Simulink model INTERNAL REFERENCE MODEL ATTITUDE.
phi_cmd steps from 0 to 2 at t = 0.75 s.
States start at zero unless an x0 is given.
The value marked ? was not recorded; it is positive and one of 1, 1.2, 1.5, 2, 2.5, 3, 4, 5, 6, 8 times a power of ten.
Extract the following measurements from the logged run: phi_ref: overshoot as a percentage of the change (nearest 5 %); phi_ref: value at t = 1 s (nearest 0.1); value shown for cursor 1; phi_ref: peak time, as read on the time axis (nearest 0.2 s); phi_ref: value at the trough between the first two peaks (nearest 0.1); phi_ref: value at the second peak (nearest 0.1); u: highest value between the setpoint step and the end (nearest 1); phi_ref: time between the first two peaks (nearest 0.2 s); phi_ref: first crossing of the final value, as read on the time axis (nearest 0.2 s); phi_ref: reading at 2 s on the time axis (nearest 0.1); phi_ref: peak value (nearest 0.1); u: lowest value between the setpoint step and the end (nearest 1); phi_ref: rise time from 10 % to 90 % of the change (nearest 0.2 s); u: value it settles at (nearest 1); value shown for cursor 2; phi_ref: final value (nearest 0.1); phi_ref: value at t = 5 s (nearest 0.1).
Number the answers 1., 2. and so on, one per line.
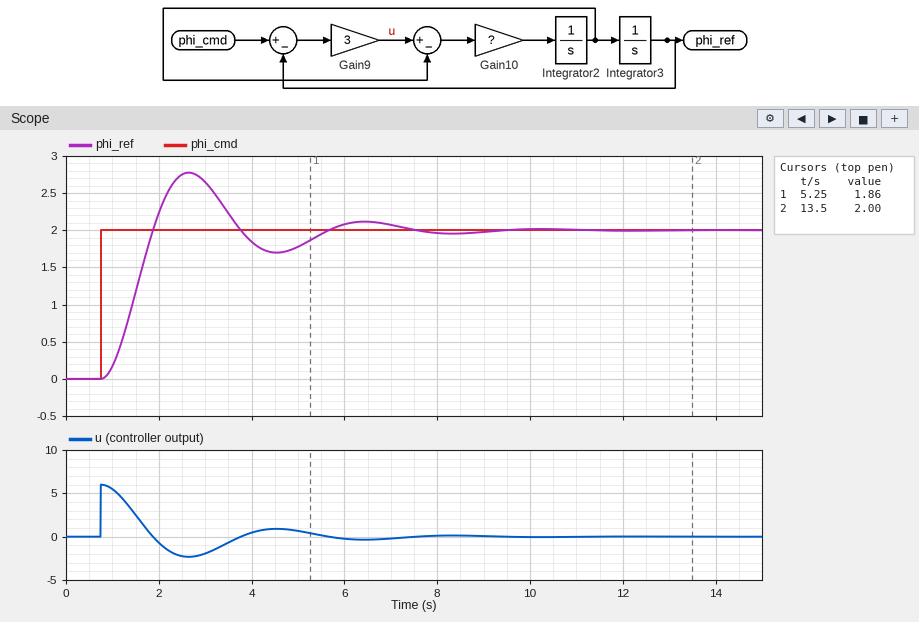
1. 40 %
2. 0.2
3. 1.86
4. 2.6 s
5. 1.7
6. 2.1
7. 6
8. 3.8 s
9. 1.8 s
10. 2.2
11. 2.8
12. -2
13. 0.8 s
14. 0
15. 2.00
16. 2.0
17. 1.8
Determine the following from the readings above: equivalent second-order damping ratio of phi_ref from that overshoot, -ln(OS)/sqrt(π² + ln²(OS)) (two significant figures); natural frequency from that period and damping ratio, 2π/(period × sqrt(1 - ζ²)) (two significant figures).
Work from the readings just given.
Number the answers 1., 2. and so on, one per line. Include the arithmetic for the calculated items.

1. ln(0.4) = -0.916; 0.916 / sqrt(9.870 + 0.840) = 0.28
2. 2π / (3.8 × sqrt(1 - 0.28²)) = 1.7 rad/s
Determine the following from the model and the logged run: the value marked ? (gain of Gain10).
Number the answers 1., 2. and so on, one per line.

1. 1
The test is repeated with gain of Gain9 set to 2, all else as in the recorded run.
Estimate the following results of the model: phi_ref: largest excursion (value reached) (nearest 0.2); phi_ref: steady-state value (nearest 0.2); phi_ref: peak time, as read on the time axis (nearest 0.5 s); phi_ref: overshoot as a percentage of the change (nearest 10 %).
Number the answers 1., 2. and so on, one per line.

1. 2.6
2. 2.0
3. 3.0 s
4. 30 %
